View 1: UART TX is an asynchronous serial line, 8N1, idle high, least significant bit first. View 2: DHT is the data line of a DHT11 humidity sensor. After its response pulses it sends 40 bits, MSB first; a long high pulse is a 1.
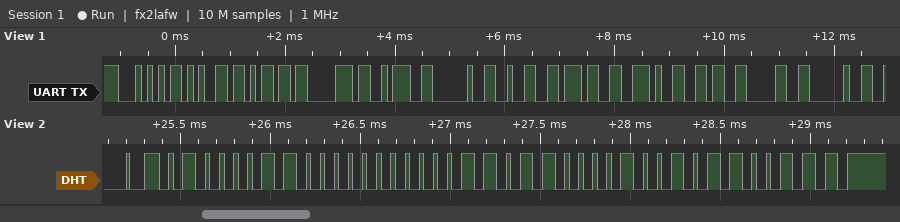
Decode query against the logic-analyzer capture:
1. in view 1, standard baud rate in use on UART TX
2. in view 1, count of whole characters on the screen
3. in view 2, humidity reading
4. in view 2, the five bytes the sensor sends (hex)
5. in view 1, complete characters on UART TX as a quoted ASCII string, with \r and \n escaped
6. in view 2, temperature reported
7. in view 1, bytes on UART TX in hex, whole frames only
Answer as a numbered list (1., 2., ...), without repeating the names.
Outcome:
1. 9600 baud
2. 12
3. 67 %
4. 43 00 1B 09 67
5. "Temp: 27.60 "
6. 27.9 °C
7. 54 65 6D 70 3A 20 32 37 2E 36 30 20
